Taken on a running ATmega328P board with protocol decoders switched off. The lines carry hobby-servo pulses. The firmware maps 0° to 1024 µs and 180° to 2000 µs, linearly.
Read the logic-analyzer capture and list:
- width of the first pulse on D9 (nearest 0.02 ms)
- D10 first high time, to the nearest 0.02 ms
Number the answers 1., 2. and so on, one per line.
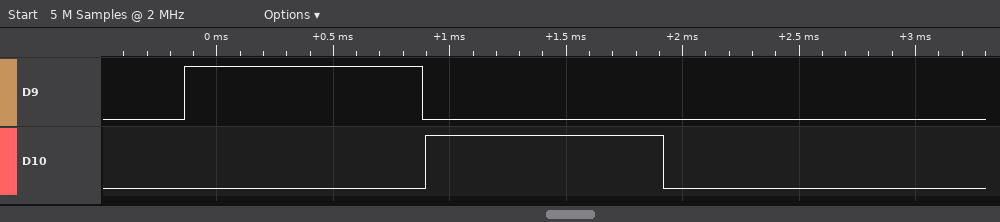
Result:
1. 1.02 ms
2. 1.02 ms
